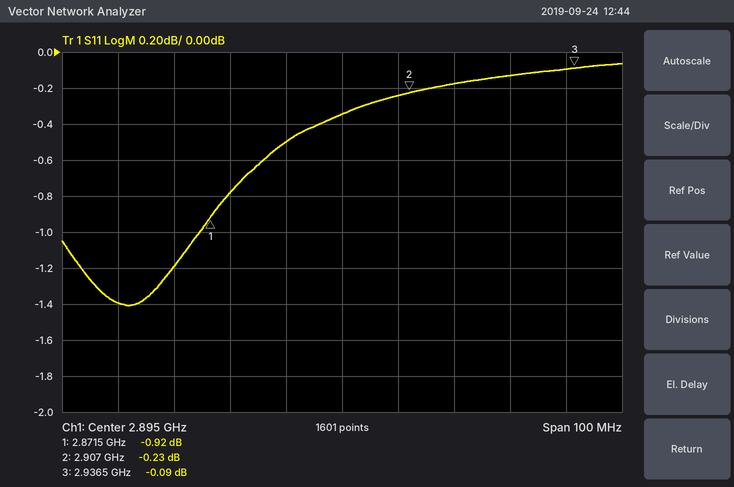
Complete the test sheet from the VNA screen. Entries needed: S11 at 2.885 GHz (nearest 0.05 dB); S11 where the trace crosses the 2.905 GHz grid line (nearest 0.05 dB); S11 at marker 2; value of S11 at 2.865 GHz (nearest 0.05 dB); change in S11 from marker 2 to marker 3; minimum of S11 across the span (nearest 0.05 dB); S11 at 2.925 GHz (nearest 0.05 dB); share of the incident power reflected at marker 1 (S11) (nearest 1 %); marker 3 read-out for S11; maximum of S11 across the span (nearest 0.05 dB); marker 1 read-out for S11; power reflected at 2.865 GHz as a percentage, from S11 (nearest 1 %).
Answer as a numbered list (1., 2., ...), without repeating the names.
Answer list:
1. -0.50 dB
2. -0.25 dB
3. -0.23 dB
4. -1.20 dB
5. 0.14 dB
6. -1.40 dB
7. -0.15 dB
8. 81 %
9. -0.09 dB
10. -0.05 dB
11. -0.92 dB
12. 76 %
